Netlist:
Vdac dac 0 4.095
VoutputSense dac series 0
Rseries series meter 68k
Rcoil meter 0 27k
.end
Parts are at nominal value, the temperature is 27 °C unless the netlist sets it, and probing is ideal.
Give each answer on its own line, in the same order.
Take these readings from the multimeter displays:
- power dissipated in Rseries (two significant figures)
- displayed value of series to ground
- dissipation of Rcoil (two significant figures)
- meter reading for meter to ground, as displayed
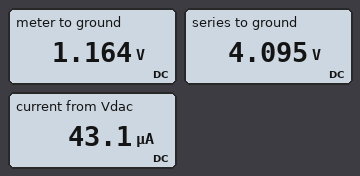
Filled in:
130 µW
4.095 V
50 µW
1.164 V
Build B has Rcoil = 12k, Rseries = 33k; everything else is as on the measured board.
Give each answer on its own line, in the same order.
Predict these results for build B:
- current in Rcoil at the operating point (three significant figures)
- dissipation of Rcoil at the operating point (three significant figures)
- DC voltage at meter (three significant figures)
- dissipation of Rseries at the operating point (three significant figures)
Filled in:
91.0 µA
99.4 µW
1.09 V
273 µW
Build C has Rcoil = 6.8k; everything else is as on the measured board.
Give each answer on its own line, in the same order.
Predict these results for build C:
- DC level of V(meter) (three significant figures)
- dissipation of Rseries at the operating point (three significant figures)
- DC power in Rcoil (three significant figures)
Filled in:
372 mV
204 µW
20.4 µW
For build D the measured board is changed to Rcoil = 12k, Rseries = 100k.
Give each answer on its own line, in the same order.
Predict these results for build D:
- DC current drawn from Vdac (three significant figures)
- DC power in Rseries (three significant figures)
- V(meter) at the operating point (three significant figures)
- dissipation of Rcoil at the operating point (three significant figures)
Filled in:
36.6 µA
134 µW
439 mV
16.0 µW
